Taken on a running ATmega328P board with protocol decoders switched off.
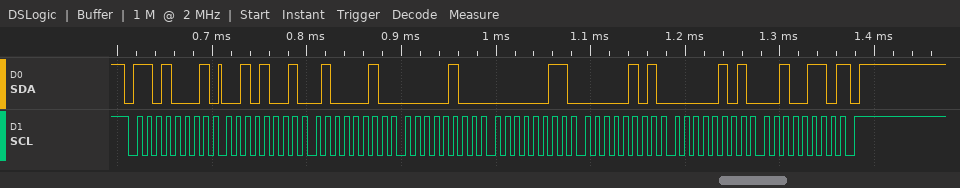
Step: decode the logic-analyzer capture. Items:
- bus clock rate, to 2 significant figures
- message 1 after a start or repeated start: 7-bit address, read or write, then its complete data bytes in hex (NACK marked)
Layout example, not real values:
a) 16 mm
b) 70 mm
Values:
a) 100 kHz
b) 0x68 read: 29 42 04 03 05 05 26 NACK
